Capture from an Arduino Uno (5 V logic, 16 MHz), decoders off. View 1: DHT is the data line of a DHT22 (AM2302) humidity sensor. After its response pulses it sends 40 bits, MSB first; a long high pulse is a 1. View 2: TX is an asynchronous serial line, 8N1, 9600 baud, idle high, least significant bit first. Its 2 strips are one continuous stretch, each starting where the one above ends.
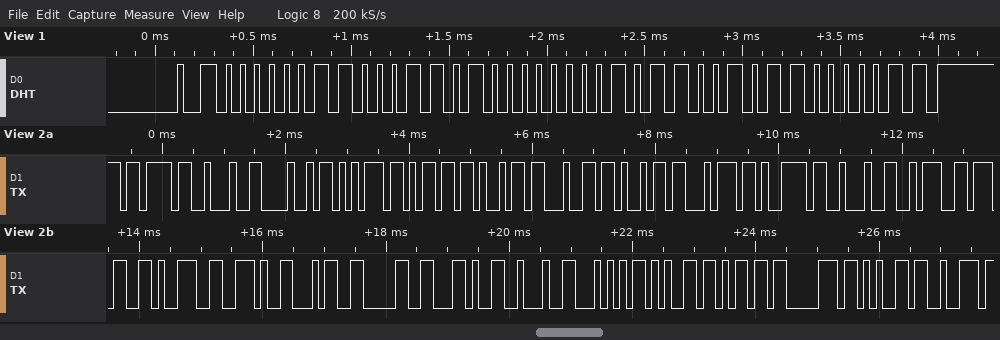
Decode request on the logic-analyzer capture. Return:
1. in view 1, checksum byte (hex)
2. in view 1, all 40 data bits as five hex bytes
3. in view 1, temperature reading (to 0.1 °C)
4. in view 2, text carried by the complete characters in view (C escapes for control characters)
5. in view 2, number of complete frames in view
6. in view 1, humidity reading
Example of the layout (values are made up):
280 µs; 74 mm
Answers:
0x83; 03 1A 01 65 83; 35.7 °C; "{\"Humidity\":79.40,\"Temper"; 25; 79.4 %
